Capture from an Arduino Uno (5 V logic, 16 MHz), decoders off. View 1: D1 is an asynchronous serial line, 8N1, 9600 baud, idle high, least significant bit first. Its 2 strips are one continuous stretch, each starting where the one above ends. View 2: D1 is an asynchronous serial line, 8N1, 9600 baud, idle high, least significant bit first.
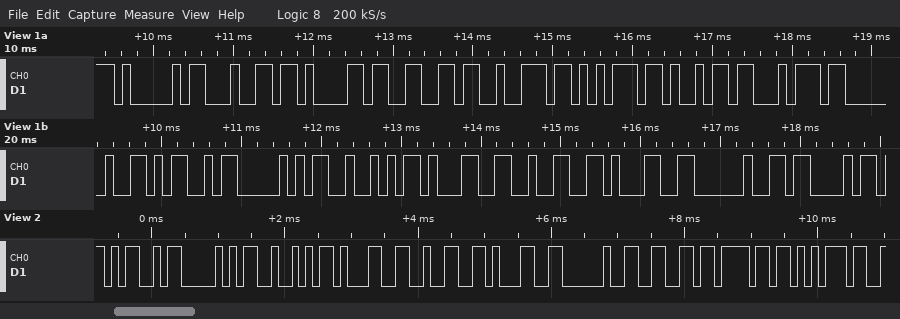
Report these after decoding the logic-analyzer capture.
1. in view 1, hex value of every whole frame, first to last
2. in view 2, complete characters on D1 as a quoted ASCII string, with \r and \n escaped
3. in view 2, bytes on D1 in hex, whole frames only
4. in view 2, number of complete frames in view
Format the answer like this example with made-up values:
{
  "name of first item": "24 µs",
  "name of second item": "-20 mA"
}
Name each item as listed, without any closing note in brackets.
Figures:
{
  "in view 1, hex value of every whole frame, first to last": "0x41 0x64 0x61 0x66 0x72 0x75 0x69 0x74 0x20 0x4D 0x50 0x52 0x31 0x32 0x31 0x20 0x43",
  "in view 2, complete characters on D1 as a quoted ASCII string, with \\r and \\n escaped": "\"MPR121 fou\"",
  "in view 2, bytes on D1 in hex, whole frames only": "4D 50 52 31 32 31 20 66 6F 75",
  "in view 2, number of complete frames in view": "10"
}
